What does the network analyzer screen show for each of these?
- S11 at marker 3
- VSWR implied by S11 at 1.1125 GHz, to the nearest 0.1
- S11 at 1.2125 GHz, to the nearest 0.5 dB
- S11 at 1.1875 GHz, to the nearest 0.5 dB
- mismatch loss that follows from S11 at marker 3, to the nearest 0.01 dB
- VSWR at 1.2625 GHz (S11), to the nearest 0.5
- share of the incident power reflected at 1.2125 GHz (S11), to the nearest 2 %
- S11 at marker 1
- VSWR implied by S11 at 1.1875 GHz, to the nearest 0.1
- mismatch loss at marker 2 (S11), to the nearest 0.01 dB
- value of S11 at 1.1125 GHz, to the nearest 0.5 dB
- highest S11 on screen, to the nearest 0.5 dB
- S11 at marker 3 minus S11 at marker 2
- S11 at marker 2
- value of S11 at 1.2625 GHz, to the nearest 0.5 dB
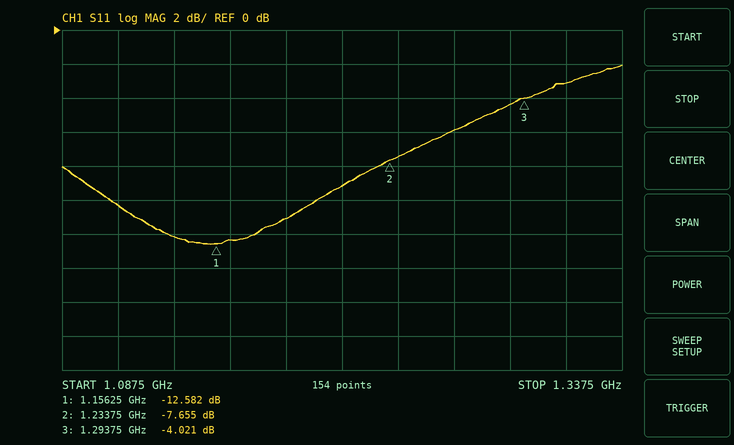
-4.021 dB
1.9
-9.0 dB
-11.0 dB
2.19 dB
3.0
12 %
-12.582 dB
1.8
0.82 dB
-10.5 dB
-2.0 dB
3.634 dB
-7.655 dB
-6.0 dB
